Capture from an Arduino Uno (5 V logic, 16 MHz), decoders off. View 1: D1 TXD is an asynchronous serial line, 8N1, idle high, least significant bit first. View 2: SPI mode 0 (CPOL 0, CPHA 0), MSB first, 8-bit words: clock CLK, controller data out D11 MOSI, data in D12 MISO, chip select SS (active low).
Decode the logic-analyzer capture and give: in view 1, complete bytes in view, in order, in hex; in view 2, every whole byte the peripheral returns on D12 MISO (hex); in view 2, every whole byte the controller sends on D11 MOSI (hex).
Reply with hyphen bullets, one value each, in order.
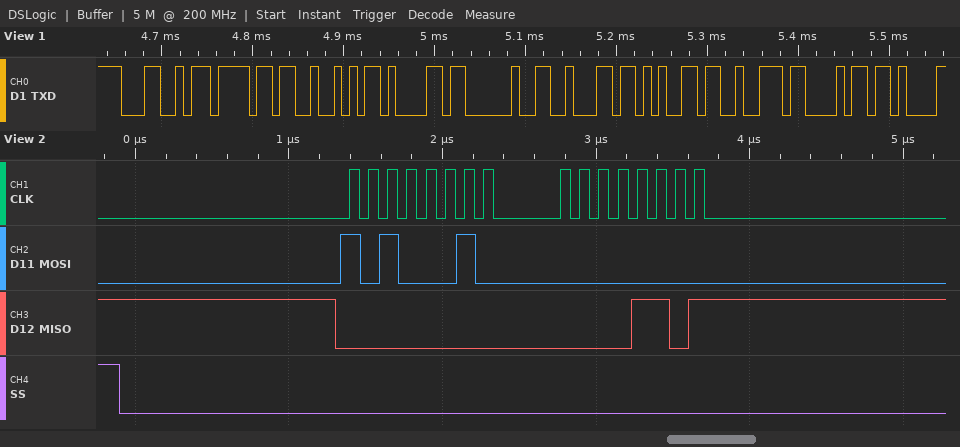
- 4C 6F 52 61 20 62 65 72 68
- 0x00 0x0D
- 0xA2 0x00
